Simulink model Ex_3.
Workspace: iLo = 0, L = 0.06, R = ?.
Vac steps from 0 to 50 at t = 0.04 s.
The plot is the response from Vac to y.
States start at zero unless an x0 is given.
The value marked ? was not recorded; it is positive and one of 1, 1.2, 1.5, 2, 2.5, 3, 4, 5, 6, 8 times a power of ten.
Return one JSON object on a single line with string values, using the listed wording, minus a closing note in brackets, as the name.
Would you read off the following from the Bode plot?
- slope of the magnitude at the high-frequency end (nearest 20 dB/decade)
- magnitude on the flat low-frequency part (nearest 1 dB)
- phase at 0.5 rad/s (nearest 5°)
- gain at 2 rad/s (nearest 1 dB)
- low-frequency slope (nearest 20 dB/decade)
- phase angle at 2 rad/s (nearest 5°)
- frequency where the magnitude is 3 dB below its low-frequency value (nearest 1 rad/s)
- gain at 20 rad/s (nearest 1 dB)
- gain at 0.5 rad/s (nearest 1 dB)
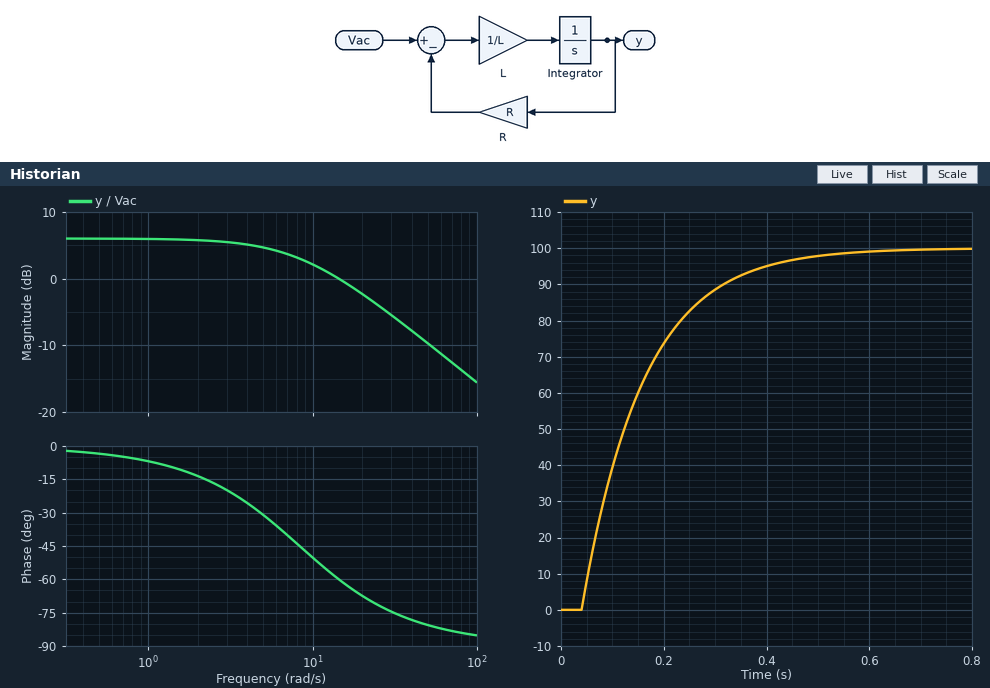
{"slope of the magnitude at the high-frequency end": "-20 dB/decade", "magnitude on the flat low-frequency part": "6 dB", "phase at 0.5 rad/s": "-5°", "gain at 2 rad/s": "6 dB", "low-frequency slope": "0 dB/decade", "phase angle at 2 rad/s": "-15°", "frequency where the magnitude is 3 dB below its low-frequency value": "8 rad/s", "gain at 20 rad/s": "-2 dB", "gain at 0.5 rad/s": "6 dB"}
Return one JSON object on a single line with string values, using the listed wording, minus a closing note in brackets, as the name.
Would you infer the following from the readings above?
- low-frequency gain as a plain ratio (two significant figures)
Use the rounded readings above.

{"low-frequency gain as a plain ratio": "2.0"}
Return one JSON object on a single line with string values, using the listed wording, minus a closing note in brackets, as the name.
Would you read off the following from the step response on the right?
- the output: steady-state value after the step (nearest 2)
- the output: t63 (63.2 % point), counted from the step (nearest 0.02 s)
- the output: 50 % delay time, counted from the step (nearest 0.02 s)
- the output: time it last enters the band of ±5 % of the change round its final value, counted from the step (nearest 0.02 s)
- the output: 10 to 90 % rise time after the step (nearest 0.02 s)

{"the output: steady-state value after the step": "100", "the output: t63 (63.2 % point), counted from the step": "0.12 s", "the output: 50 % delay time, counted from the step": "0.08 s", "the output: time it last enters the band of ±5 % of the change round its final value, counted from the step": "0.36 s", "the output: 10 to 90 % rise time after the step": "0.26 s"}
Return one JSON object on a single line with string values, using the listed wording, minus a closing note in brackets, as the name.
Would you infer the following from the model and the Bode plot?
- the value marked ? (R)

{"the value marked ?": "0.5"}
